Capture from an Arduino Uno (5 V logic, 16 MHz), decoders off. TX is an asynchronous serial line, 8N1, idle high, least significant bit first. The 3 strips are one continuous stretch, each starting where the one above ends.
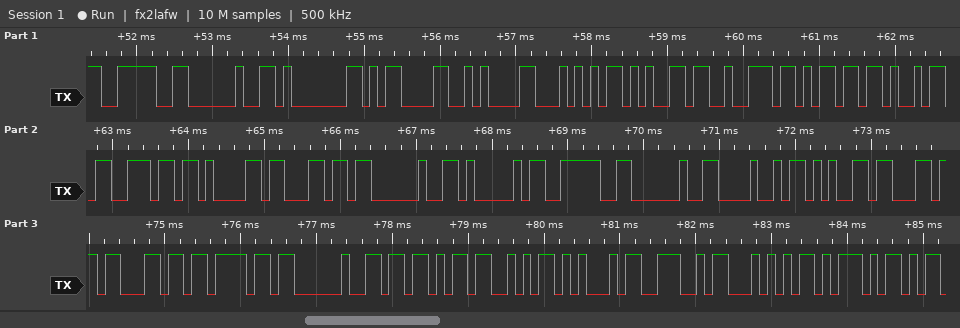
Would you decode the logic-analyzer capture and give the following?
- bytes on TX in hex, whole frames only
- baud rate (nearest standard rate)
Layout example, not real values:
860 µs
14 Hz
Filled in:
3E 20 01 0D 0A 54 65 72 6D 69 6E 61 6C 20 41 3E 20 48 65 6C 6C 6F 20 5B 53 45 4E 54 5D
9600 baud
